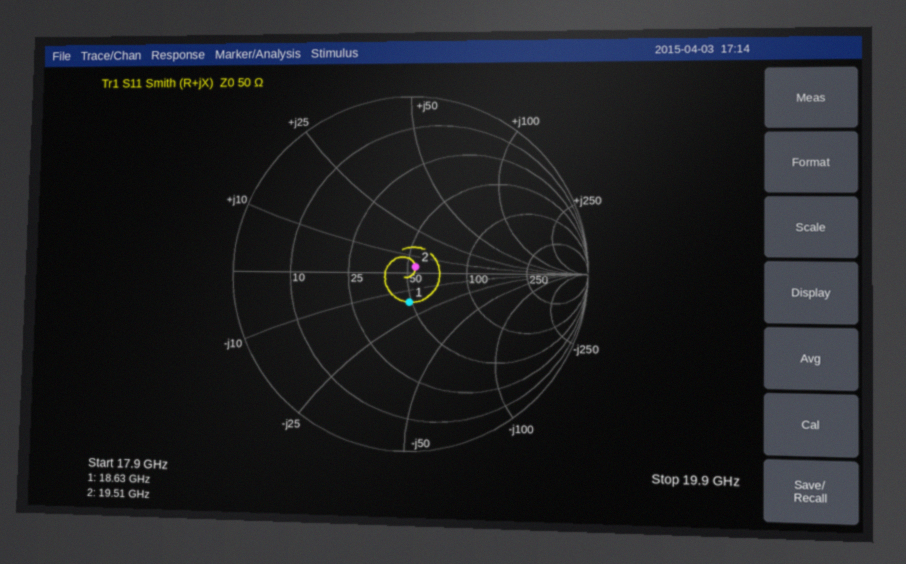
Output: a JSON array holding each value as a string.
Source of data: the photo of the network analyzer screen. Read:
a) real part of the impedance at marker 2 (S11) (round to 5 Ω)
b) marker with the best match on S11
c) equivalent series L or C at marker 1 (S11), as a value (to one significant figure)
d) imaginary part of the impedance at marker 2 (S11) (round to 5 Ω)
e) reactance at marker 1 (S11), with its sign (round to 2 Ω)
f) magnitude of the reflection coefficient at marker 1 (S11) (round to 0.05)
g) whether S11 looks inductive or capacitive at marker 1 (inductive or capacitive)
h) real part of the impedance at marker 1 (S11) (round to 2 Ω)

["55 Ω", "marker 2", "500 fF", "+5 Ω", "-16 Ω", "0.15", "capacitive", "48 Ω"]
